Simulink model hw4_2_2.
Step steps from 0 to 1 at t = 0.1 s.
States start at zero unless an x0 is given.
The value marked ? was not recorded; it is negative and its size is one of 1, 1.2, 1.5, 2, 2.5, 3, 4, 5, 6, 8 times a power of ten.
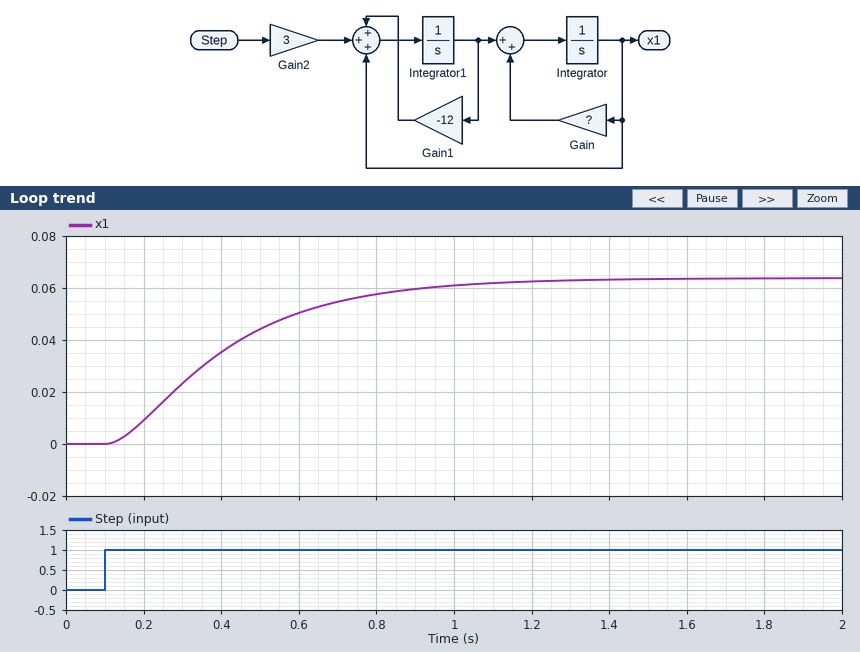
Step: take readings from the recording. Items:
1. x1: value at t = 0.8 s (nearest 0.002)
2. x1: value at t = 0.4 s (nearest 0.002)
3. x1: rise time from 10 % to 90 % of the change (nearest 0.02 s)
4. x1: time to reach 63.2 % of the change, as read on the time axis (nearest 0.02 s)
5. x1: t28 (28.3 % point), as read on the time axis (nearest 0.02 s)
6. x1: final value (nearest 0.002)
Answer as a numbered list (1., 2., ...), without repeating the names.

1. 0.058
2. 0.036
3. 0.62 s
4. 0.46 s
5. 0.26 s
6. 0.064
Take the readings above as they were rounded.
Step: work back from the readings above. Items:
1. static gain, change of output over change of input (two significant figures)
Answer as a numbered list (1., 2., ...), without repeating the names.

1. 0.064
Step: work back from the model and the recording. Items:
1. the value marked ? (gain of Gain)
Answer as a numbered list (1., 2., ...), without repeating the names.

1. -4
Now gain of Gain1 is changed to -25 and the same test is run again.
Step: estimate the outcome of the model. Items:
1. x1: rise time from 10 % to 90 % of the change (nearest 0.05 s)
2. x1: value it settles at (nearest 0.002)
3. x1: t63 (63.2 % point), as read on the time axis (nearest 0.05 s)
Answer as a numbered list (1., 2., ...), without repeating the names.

1. 0.55 s
2. 0.030
3. 0.40 s
